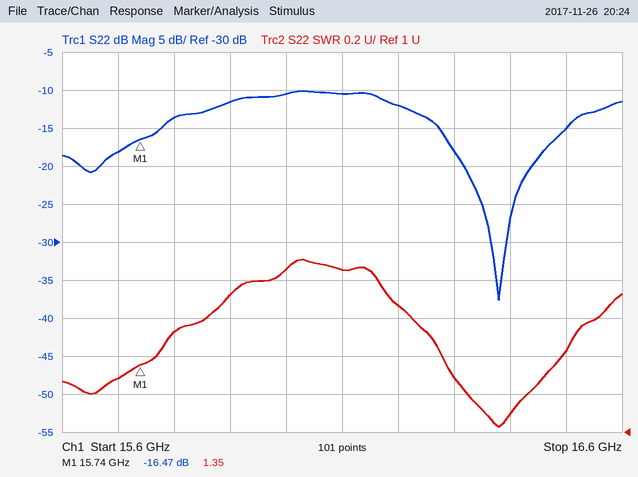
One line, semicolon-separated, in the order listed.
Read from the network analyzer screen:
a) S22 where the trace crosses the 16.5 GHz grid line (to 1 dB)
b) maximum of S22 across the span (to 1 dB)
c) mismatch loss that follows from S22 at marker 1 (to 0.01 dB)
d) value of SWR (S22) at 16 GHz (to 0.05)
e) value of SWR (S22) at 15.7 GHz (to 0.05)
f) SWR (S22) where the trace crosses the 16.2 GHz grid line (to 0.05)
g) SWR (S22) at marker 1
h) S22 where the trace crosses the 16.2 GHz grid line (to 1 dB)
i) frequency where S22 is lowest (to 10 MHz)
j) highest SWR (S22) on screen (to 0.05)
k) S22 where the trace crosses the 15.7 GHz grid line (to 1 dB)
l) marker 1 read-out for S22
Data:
-15 dB; -10 dB; 0.10 dB; 1.85; 1.30; 1.65; 1.35; -12 dB; 16.38 GHz; 1.90; -18 dB; -16.47 dB
